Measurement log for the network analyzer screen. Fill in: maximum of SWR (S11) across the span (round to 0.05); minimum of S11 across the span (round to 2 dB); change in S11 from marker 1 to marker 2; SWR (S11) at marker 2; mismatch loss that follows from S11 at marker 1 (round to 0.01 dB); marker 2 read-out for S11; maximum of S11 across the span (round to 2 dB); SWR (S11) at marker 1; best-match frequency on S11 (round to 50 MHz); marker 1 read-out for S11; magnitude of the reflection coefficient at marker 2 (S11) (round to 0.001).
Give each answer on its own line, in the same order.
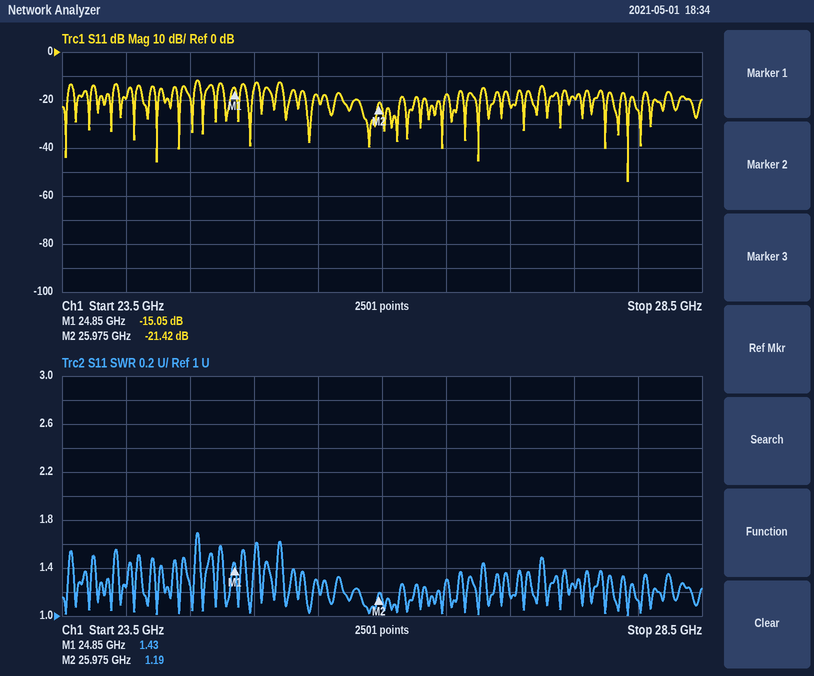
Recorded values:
1.70
-54 dB
-6.37 dB
1.19
0.14 dB
-21.42 dB
-12 dB
1.43
27.90 GHz
-15.05 dB
0.085
